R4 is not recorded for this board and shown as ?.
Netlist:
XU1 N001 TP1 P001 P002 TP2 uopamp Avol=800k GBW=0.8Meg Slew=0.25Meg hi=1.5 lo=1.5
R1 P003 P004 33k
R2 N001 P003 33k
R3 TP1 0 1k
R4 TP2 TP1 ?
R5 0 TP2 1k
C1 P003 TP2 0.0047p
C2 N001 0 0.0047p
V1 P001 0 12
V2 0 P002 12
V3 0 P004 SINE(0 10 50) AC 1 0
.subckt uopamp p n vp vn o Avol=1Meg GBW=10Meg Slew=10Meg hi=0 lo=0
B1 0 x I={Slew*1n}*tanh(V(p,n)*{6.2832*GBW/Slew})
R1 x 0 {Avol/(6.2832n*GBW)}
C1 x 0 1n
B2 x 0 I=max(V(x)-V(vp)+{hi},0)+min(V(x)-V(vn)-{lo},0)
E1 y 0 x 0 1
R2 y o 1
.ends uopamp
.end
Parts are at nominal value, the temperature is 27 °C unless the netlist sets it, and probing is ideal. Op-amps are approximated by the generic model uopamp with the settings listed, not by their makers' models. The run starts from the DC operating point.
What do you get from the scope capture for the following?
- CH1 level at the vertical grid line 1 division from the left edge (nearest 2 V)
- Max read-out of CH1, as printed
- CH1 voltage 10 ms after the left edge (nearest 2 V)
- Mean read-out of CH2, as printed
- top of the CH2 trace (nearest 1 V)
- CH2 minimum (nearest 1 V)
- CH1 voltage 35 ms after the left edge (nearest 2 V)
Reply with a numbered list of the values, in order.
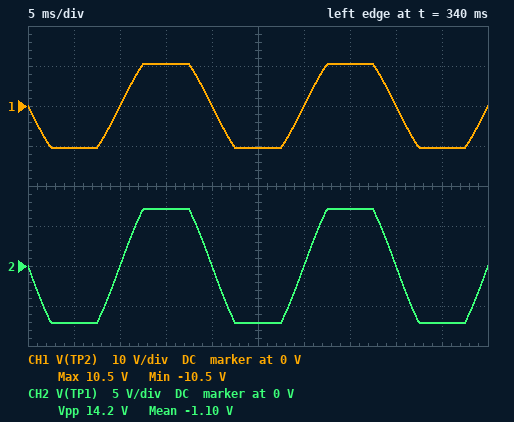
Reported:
1. -10 V
2. 10.5 V
3. 0 V
4. -1.10 V
5. 7 V
6. -7 V
7. 10 V
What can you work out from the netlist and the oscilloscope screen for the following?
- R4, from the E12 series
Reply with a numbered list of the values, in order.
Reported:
1. 470 Ω
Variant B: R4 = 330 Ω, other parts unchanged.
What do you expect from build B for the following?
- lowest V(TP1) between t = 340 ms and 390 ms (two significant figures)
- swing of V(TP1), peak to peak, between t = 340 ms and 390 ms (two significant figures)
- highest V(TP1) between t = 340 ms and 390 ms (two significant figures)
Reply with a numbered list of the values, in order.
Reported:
1. -7.9 V
2. 16 V
3. 7.9 V
